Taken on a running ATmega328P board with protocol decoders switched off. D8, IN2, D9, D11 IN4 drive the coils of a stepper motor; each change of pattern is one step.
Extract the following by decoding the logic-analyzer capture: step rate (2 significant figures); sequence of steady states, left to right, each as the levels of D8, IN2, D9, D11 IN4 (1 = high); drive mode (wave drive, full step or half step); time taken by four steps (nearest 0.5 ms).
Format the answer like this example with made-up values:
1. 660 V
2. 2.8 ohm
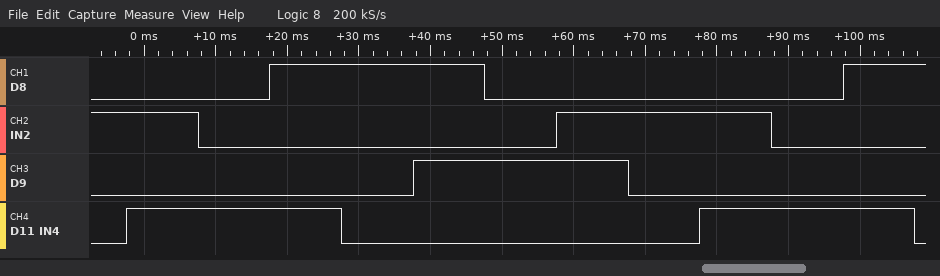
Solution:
1. 100 steps/s
2. 0100 0101 0001 1001 1000 1010 0010 0110 0100 0101 0001 1001 1000
3. half step
4. 40.0 ms
